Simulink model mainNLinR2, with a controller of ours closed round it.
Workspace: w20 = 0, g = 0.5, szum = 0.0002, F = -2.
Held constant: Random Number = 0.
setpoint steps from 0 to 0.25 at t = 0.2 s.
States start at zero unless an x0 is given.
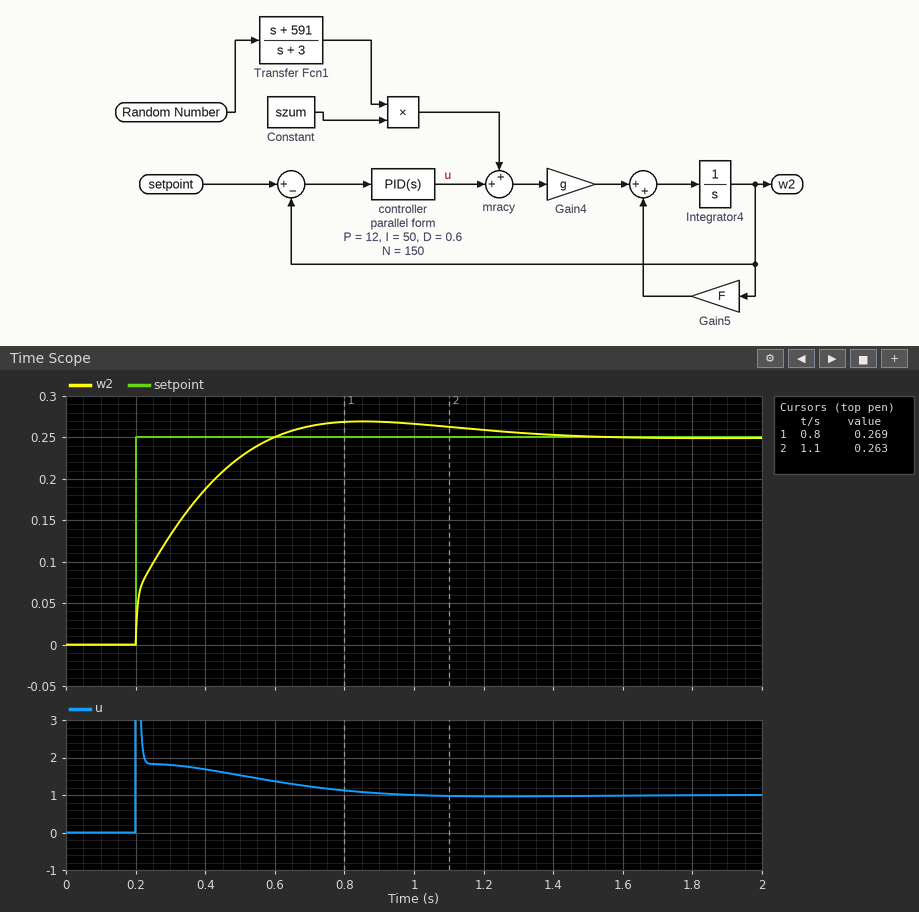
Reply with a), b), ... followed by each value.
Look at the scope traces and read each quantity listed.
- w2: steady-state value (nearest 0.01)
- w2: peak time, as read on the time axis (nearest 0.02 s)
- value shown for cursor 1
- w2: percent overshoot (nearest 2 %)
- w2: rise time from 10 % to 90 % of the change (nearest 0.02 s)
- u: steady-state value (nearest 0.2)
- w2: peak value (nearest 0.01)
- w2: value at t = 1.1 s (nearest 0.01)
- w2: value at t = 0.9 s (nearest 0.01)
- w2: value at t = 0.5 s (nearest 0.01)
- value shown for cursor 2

a) 0.25
b) 0.86 s
c) 0.269
d) 8 %
e) 0.30 s
f) 1.0
g) 0.27
h) 0.26
i) 0.27
j) 0.23
k) 0.263
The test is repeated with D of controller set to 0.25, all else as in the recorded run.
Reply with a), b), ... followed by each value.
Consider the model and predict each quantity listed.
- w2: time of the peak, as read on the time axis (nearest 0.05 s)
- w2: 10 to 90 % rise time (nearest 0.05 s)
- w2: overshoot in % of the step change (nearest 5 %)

a) 0.80 s
b) 0.25 s
c) 10 %
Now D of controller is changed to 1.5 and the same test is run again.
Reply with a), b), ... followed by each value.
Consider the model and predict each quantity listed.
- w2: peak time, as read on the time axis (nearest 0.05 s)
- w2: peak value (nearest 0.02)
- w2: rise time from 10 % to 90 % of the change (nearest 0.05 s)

a) 1.00 s
b) 0.26
c) 0.35 s
